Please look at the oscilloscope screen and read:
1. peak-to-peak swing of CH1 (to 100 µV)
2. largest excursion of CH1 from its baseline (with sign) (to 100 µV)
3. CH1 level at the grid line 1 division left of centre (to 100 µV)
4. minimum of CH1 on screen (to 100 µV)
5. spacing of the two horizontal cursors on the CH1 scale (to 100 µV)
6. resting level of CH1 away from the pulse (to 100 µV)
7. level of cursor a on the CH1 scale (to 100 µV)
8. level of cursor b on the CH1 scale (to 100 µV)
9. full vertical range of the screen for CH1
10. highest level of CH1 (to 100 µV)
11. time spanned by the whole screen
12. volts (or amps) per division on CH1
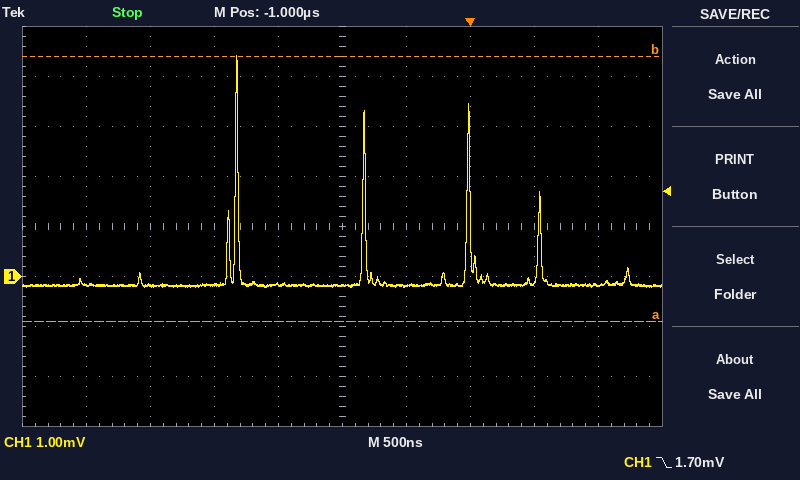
4.6 mV
+4.6 mV
-200 µV
-200 µV
5.3 mV
-200 µV
-900 µV
4.4 mV
8 mV
4.4 mV
5 µs
1 mV
